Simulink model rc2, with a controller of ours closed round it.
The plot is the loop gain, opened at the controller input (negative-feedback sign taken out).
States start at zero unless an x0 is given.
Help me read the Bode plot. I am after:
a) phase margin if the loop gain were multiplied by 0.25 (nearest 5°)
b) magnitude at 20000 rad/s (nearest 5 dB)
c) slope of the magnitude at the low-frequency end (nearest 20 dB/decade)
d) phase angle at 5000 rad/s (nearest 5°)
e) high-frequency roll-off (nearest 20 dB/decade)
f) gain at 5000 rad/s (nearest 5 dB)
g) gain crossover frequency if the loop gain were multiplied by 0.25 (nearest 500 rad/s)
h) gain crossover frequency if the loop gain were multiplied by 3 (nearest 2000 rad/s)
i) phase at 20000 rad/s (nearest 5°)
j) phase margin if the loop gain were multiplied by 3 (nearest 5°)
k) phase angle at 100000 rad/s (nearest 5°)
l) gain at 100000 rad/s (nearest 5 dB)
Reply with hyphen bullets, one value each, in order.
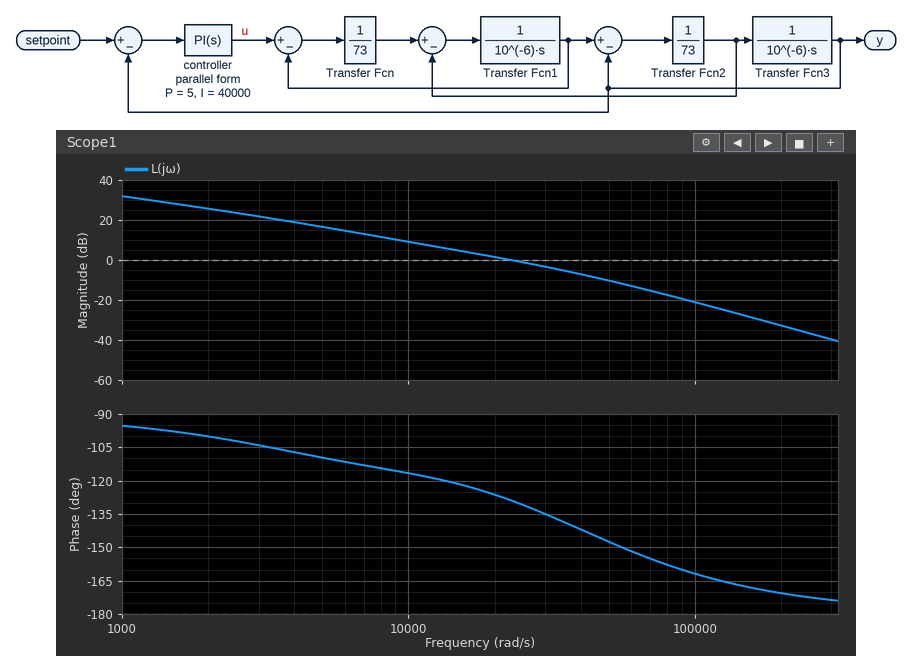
- 65°
- 0 dB
- -20 dB/decade
- -110°
- -40 dB/decade
- 15 dB
- 7500 rad/s
- 48000 rad/s
- -125°
- 35°
- -160°
- -20 dB
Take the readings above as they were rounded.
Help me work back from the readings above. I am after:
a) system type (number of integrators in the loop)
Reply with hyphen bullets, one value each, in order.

- 1
